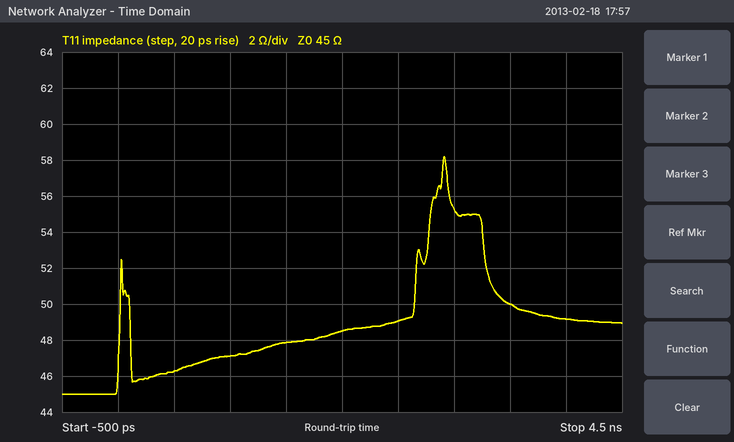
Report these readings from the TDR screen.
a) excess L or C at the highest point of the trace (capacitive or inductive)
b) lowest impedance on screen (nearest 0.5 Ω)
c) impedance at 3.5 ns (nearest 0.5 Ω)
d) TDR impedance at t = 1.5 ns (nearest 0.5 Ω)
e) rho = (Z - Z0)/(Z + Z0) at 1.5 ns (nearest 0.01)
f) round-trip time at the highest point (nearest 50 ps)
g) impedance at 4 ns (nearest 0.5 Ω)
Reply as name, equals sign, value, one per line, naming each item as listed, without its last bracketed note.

excess L or C at the highest point of the trace = inductive
lowest impedance on screen = 45.0 Ω
impedance at 3.5 ns = 50.0 Ω
TDR impedance at t = 1.5 ns = 48.0 Ω
rho = (Z - Z0)/(Z + Z0) at 1.5 ns = +0.03
round-trip time at the highest point = 2.90 ns
impedance at 4 ns = 49.0 Ω
